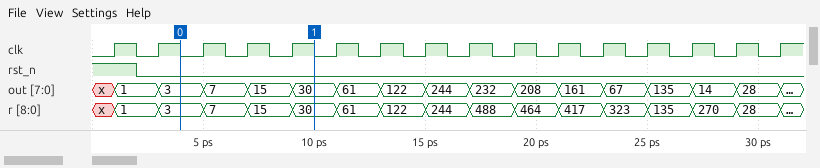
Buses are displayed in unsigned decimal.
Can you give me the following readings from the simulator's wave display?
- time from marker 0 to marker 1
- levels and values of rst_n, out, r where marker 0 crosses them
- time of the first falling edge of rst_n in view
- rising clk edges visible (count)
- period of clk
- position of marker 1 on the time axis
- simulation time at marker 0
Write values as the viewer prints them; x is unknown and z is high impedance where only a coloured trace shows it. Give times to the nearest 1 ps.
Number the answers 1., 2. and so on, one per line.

1. 6 ps
2. rst_n=0, out=3, r=3
3. 2 ps
4. 16
5. 2 ps
6. 10 ps
7. 4 ps
